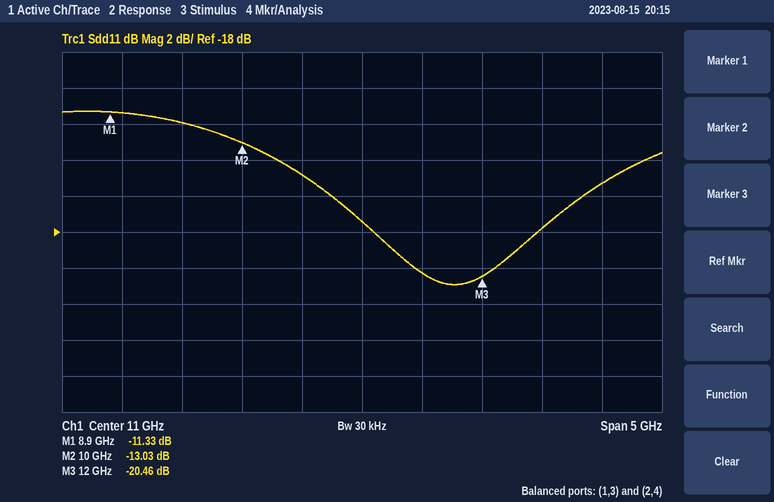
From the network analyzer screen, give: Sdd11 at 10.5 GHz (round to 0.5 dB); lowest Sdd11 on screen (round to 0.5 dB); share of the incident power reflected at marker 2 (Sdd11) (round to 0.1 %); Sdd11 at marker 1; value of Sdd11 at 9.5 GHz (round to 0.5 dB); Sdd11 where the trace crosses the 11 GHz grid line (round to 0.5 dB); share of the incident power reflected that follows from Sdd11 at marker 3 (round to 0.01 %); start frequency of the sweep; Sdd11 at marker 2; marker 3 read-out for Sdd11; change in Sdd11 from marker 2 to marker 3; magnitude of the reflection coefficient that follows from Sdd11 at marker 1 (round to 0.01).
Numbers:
-15.0 dB
-21.0 dB
5.0 %
-11.33 dB
-12.0 dB
-17.5 dB
0.90 %
8.5 GHz
-13.03 dB
-20.46 dB
-7.43 dB
0.27
